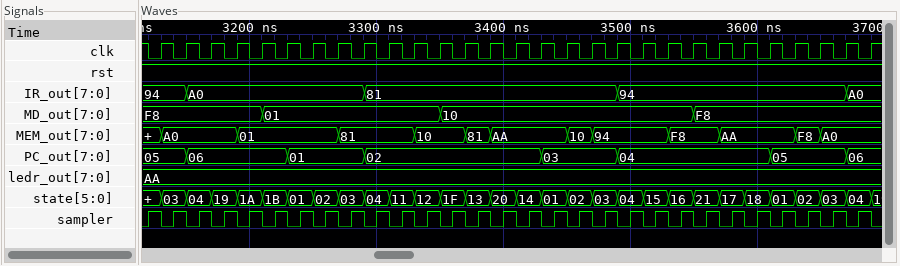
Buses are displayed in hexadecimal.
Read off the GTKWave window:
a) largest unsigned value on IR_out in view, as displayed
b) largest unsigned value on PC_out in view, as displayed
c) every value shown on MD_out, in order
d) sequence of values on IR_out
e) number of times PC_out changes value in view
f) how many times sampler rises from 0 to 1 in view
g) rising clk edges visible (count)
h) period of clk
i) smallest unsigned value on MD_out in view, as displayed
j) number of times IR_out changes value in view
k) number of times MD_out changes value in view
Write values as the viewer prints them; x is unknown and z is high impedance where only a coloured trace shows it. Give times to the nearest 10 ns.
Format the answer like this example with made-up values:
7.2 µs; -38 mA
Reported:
A0; 06; F8, 01, 10, F8; 94, A0, 81, 94, A0; 7; 29; 29; 20 ns; 01; 4; 3
